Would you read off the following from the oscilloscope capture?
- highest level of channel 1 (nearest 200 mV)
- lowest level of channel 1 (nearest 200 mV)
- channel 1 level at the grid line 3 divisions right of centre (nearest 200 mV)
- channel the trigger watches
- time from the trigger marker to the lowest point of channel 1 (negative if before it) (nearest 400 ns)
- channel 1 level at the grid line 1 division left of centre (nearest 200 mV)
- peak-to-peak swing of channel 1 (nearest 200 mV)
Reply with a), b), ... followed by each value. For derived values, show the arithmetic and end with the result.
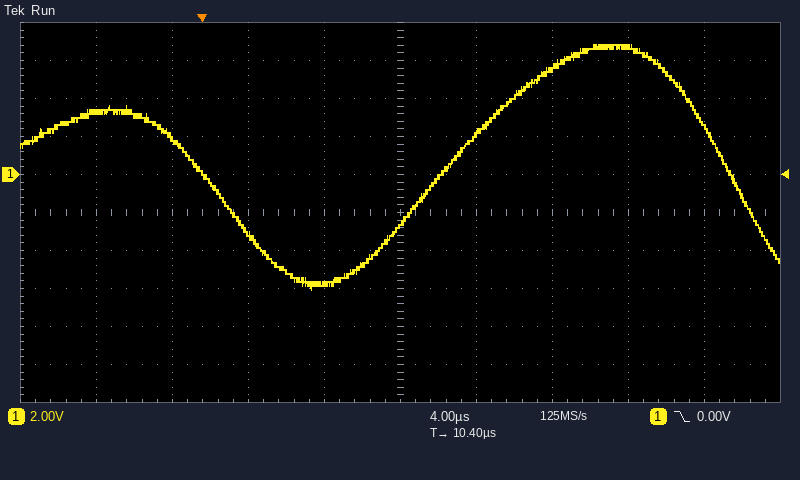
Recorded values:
a) 6.8 V
b) -6.0 V
c) 6.8 V
d) channel 1
e) +5.6 µs
f) -5.8 V
g) 6.8 V − (-6.0 V) = 12.8 V
